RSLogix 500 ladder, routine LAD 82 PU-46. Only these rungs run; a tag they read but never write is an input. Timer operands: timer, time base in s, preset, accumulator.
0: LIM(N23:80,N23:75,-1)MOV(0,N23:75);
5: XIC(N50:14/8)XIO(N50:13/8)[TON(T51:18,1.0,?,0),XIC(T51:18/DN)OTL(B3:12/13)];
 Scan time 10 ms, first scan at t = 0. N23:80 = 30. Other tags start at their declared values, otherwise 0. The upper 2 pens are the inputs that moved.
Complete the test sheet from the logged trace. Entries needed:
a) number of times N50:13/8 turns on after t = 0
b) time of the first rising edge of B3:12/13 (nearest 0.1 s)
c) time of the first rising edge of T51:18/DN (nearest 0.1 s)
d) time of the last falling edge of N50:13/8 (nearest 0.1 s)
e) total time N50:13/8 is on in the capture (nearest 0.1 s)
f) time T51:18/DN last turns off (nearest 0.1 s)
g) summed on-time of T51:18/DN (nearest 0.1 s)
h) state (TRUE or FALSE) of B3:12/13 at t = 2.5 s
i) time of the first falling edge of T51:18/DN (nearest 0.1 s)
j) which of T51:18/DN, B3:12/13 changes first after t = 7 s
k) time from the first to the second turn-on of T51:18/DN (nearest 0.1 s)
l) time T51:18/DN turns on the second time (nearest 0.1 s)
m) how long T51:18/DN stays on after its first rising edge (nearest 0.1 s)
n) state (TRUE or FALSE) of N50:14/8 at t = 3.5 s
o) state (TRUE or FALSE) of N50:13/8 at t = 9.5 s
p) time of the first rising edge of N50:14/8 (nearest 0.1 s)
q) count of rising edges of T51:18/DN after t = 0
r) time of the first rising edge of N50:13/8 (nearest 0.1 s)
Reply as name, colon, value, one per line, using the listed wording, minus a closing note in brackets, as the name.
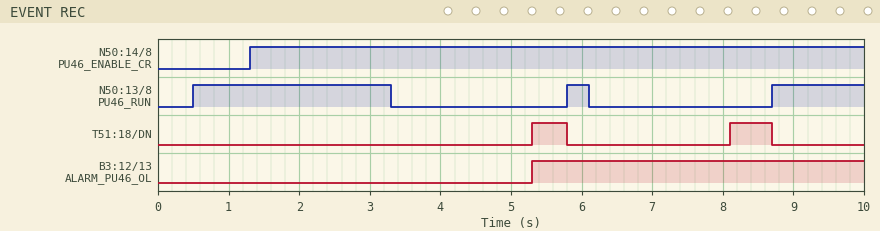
number of times N50:13/8 turns on after t = 0: 3
time of the first rising edge of B3:12/13: 5.3 s
time of the first rising edge of T51:18/DN: 5.3 s
time of the last falling edge of N50:13/8: 6.1 s
total time N50:13/8 is on in the capture: 4.4 s
time T51:18/DN last turns off: 8.7 s
summed on-time of T51:18/DN: 1.1 s
state (TRUE or FALSE) of B3:12/13 at t = 2.5 s: FALSE
time of the first falling edge of T51:18/DN: 5.8 s
which of T51:18/DN, B3:12/13 changes first after t = 7 s: T51:18/DN
time from the first to the second turn-on of T51:18/DN: 2.8 s
time T51:18/DN turns on the second time: 8.1 s
how long T51:18/DN stays on after its first rising edge: 0.5 s
state (TRUE or FALSE) of N50:14/8 at t = 3.5 s: TRUE
state (TRUE or FALSE) of N50:13/8 at t = 9.5 s: TRUE
time of the first rising edge of N50:14/8: 1.3 s
count of rising edges of T51:18/DN after t = 0: 2
time of the first rising edge of N50:13/8: 0.5 s
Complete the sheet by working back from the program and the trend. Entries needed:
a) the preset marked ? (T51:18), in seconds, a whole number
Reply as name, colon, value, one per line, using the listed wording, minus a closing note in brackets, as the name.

the preset marked ? (T51:18), in seconds, a whole number: 2 s
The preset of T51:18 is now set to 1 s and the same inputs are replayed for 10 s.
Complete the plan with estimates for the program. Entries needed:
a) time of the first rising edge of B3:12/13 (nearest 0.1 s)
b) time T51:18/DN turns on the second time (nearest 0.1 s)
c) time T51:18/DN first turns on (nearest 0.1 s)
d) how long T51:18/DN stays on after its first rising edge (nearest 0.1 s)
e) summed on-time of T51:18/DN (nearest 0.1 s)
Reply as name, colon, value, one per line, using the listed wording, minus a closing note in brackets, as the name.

time of the first rising edge of B3:12/13: 4.3 s
time T51:18/DN turns on the second time: 7.1 s
time T51:18/DN first turns on: 4.3 s
how long T51:18/DN stays on after its first rising edge: 1.5 s
summed on-time of T51:18/DN: 3.1 s
